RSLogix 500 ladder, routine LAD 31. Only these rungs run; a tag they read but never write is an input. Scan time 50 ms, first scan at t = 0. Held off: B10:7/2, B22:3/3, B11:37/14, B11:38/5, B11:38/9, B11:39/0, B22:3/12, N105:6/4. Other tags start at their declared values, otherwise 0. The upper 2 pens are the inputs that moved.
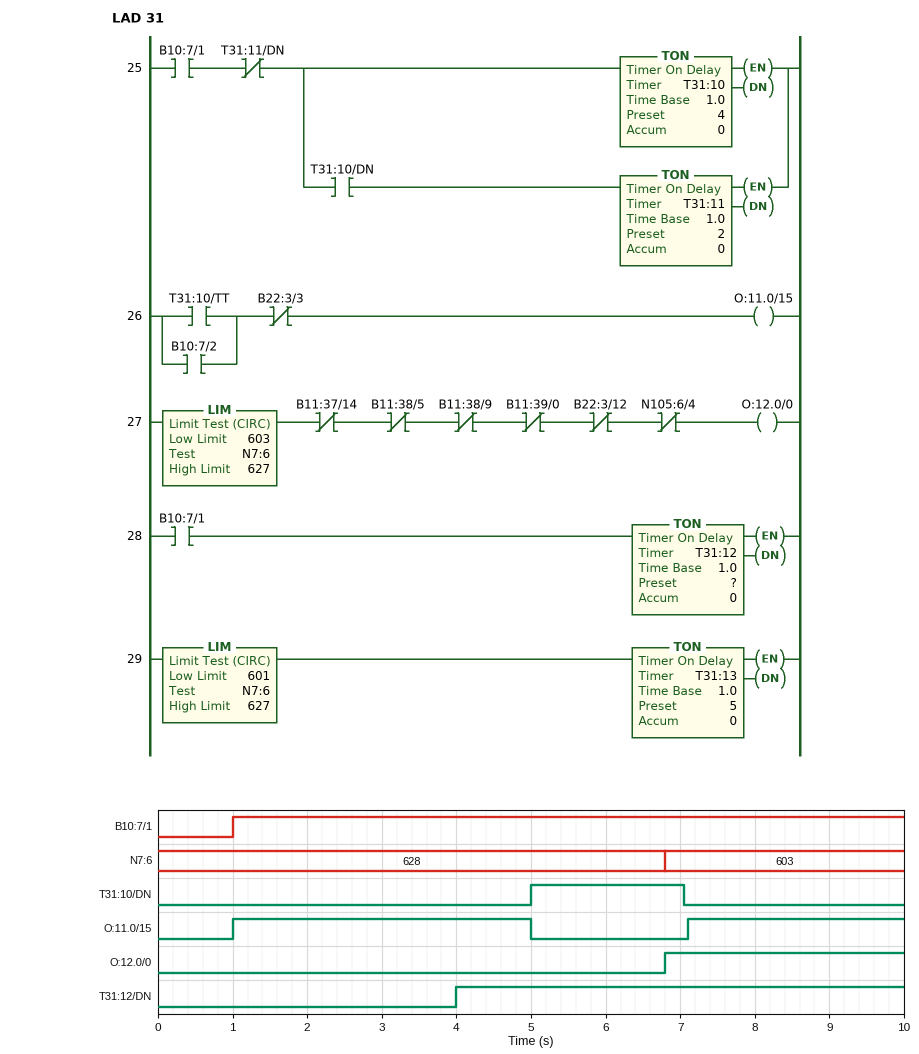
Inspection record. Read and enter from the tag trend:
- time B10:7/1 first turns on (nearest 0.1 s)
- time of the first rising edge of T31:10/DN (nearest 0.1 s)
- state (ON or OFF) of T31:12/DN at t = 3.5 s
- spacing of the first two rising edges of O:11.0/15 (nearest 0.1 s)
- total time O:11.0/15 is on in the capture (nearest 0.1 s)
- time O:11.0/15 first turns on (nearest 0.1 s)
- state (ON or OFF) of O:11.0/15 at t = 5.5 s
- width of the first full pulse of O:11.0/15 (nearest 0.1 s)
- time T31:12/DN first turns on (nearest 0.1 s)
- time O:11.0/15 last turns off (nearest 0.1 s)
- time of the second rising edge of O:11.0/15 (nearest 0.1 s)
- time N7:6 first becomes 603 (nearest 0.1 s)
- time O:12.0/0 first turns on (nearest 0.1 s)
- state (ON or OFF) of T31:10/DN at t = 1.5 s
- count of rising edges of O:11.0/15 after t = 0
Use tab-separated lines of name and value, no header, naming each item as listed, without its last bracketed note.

time B10:7/1 first turns on	1.0 s
time of the first rising edge of T31:10/DN	5.0 s
state (ON or OFF) of T31:12/DN at t = 3.5 s	OFF
spacing of the first two rising edges of O:11.0/15	6.1 s
total time O:11.0/15 is on in the capture	6.9 s
time O:11.0/15 first turns on	1.0 s
state (ON or OFF) of O:11.0/15 at t = 5.5 s	OFF
width of the first full pulse of O:11.0/15	4.0 s
time T31:12/DN first turns on	4.0 s
time O:11.0/15 last turns off	5.0 s
time of the second rising edge of O:11.0/15	7.1 s
time N7:6 first becomes 603	6.8 s
time O:12.0/0 first turns on	6.8 s
state (ON or OFF) of T31:10/DN at t = 1.5 s	OFF
count of rising edges of O:11.0/15 after t = 0	2
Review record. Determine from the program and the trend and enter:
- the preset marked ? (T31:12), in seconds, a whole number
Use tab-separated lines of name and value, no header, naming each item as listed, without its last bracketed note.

the preset marked ? (T31:12), in seconds, a whole number	3 s
